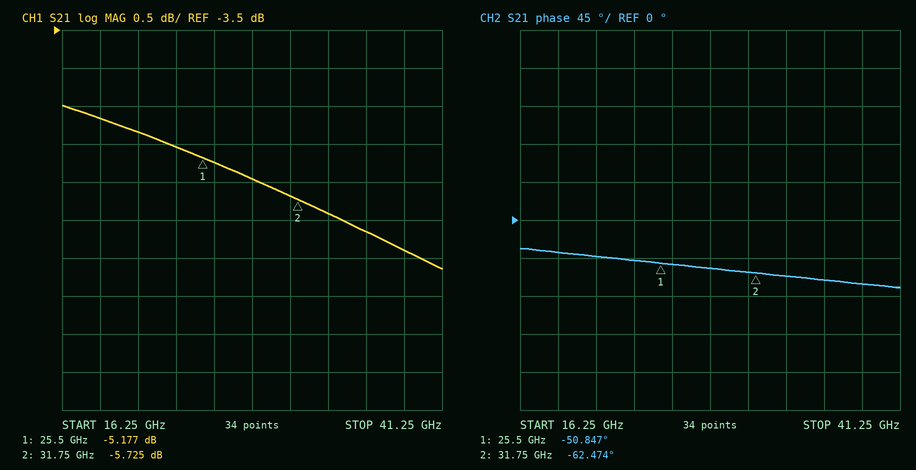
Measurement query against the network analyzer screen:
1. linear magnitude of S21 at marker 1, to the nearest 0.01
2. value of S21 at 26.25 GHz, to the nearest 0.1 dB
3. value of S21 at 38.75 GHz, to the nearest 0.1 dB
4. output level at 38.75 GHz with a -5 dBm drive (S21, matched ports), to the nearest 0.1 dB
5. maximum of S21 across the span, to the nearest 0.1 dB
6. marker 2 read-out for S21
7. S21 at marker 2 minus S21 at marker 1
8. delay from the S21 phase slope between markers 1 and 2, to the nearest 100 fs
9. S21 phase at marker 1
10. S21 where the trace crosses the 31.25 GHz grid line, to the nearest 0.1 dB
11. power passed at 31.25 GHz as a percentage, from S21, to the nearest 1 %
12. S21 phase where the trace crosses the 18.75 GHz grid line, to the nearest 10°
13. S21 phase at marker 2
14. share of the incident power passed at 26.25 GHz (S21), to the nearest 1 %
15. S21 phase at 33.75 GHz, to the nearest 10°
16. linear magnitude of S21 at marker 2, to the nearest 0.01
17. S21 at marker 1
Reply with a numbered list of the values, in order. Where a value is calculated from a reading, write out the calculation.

1. 10^(-5.177/20) ≈ 0.55
2. -5.2 dB
3. -6.4 dB
4. -5 dBm + (-6.4 dB) = -11.4 dBm
5. -4.5 dB
6. -5.725 dB
7. -5.725 − (-5.177) = -0.548 dB
8. −(-62.474° − (-50.847°))/(360° × 6.25 GHz) ≈ 5.2 ps
9. -50.847°
10. -5.7 dB
11. 10^(-5.7/10) ≈ 27 %
12. -40°
13. -62.474°
14. 10^(-5.2/10) ≈ 30 %
15. -70°
16. 10^(-5.725/20) ≈ 0.52
17. -5.177 dB
